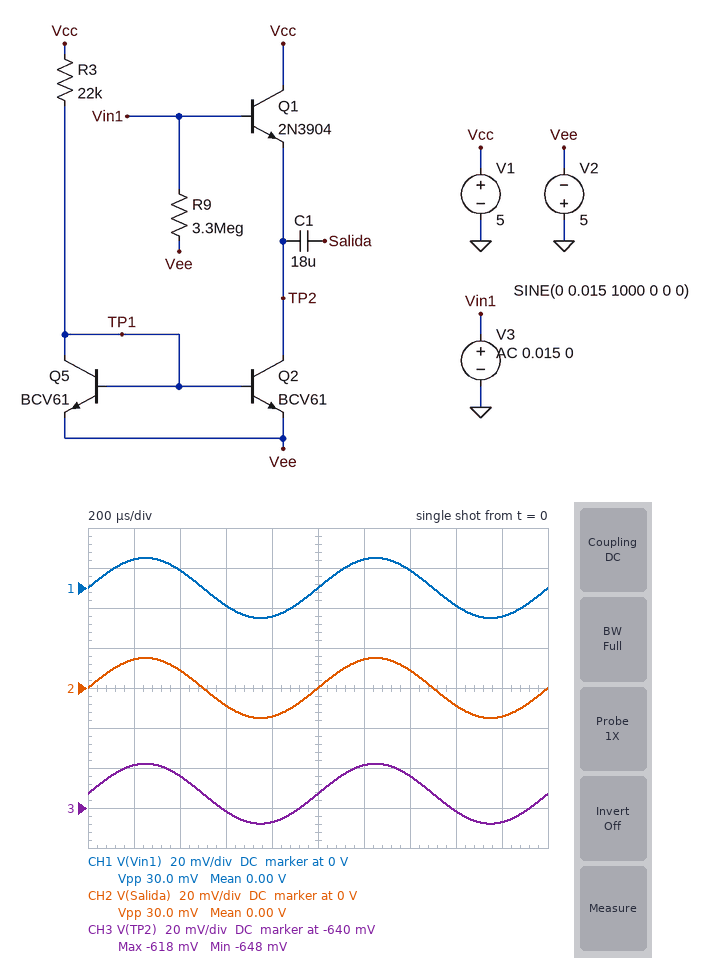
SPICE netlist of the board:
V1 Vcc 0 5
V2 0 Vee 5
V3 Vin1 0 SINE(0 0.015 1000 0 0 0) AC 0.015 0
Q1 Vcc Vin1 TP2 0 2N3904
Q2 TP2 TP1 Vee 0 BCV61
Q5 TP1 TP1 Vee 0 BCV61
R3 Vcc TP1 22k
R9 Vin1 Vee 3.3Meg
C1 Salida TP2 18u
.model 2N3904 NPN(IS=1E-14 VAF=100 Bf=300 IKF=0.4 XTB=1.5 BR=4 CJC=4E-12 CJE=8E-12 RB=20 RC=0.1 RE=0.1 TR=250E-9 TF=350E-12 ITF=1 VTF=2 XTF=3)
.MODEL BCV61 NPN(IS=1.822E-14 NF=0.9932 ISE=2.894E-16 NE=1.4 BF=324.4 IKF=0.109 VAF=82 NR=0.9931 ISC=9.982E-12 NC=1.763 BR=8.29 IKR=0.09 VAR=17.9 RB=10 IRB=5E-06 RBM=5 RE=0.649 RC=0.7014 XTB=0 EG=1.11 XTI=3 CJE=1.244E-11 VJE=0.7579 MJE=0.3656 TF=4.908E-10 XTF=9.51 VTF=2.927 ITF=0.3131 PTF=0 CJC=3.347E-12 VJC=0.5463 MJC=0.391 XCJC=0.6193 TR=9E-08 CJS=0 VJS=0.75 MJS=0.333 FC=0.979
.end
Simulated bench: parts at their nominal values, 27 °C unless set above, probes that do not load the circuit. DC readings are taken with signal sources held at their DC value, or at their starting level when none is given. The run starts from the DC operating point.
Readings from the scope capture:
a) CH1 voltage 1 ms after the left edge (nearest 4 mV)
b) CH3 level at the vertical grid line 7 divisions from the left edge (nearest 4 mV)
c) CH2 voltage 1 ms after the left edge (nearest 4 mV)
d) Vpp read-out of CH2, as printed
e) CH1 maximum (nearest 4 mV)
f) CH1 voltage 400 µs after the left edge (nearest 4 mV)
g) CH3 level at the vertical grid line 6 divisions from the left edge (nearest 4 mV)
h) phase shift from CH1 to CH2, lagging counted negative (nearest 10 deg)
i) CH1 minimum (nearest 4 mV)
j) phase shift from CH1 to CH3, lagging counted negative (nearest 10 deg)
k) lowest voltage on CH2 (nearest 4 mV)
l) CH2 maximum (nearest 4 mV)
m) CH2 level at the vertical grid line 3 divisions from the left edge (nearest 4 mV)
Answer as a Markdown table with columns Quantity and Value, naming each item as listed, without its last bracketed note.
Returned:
| Quantity | Value |
|---|---|
| CH1 voltage 1 ms after the left edge | 0 V |
| CH3 level at the vertical grid line 7 divisions from the left edge | -624 mV |
| CH2 voltage 1 ms after the left edge | 0 V |
| Vpp read-out of CH2, as printed | 30.0 mV |
| CH1 maximum | 16 mV |
| CH1 voltage 400 µs after the left edge | 8 mV |
| CH3 level at the vertical grid line 6 divisions from the left edge | -620 mV |
| phase shift from CH1 to CH2, lagging counted negative | 0 deg |
| CH1 minimum | -16 mV |
| phase shift from CH1 to CH3, lagging counted negative | 0 deg |
| lowest voltage on CH2 | -16 mV |
| CH2 maximum | 16 mV |
| CH2 level at the vertical grid line 3 divisions from the left edge | -8 mV |
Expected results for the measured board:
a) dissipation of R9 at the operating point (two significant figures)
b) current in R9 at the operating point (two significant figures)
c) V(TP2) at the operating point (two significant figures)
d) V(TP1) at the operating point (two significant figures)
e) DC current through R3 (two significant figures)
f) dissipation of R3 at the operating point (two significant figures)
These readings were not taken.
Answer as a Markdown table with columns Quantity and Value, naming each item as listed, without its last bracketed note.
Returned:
| Quantity | Value |
|---|---|
| dissipation of R9 at the operating point | 7.6 µW |
| current in R9 at the operating point | 1.5 µA |
| V(TP2) at the operating point | -630 mV |
| V(TP1) at the operating point | -4.4 V |
| DC current through R3 | 430 µA |
| dissipation of R3 at the operating point | 4.0 mW |
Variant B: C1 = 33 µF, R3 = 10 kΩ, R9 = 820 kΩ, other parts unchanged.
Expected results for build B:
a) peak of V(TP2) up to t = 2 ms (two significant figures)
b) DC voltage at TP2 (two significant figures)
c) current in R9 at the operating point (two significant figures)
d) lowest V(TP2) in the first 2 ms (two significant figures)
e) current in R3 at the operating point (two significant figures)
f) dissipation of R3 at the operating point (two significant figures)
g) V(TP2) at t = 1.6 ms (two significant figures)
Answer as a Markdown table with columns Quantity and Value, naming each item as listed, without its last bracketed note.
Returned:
| Quantity | Value |
|---|---|
| peak of V(TP2) up to t = 2 ms | -640 mV |
| DC voltage at TP2 | -650 mV |
| current in R9 at the operating point | 6.1 µA |
| lowest V(TP2) in the first 2 ms | -670 mV |
| current in R3 at the operating point | 940 µA |
| dissipation of R3 at the operating point | 8.8 mW |
| V(TP2) at t = 1.6 ms | -660 mV |
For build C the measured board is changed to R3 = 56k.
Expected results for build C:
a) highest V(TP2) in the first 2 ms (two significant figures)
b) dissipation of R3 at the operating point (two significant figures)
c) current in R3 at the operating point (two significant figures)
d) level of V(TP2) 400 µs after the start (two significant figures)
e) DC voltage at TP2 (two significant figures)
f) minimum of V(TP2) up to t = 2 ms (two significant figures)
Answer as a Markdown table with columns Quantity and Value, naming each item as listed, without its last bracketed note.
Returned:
| Quantity | Value |
|---|---|
| highest V(TP2) in the first 2 ms | -590 mV |
| dissipation of R3 at the operating point | 1.6 mW |
| current in R3 at the operating point | 170 µA |
| level of V(TP2) 400 µs after the start | -600 mV |
| DC voltage at TP2 | -610 mV |
| minimum of V(TP2) up to t = 2 ms | -620 mV |
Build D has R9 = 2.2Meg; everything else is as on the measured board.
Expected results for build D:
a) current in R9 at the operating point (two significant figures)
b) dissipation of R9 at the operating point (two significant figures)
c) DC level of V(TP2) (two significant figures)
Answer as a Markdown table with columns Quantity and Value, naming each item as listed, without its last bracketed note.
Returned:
| Quantity | Value |
|---|---|
| current in R9 at the operating point | 2.3 µA |
| dissipation of R9 at the operating point | 11 µW |
| DC level of V(TP2) | -630 mV |
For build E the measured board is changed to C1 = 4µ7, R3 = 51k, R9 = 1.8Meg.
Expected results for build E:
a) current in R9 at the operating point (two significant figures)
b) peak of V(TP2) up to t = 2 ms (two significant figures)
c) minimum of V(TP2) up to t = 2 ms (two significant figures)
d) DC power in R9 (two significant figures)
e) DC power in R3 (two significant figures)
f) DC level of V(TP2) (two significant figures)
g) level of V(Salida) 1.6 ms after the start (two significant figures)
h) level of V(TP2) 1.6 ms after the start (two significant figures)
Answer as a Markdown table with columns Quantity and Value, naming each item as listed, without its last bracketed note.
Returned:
| Quantity | Value |
|---|---|
| current in R9 at the operating point | 2.8 µA |
| peak of V(TP2) up to t = 2 ms | -600 mV |
| minimum of V(TP2) up to t = 2 ms | -630 mV |
| DC power in R9 | 14 µW |
| DC power in R3 | 1.7 mW |
| DC level of V(TP2) | -610 mV |
| level of V(Salida) 1.6 ms after the start | -8.8 mV |
| level of V(TP2) 1.6 ms after the start | -620 mV |
